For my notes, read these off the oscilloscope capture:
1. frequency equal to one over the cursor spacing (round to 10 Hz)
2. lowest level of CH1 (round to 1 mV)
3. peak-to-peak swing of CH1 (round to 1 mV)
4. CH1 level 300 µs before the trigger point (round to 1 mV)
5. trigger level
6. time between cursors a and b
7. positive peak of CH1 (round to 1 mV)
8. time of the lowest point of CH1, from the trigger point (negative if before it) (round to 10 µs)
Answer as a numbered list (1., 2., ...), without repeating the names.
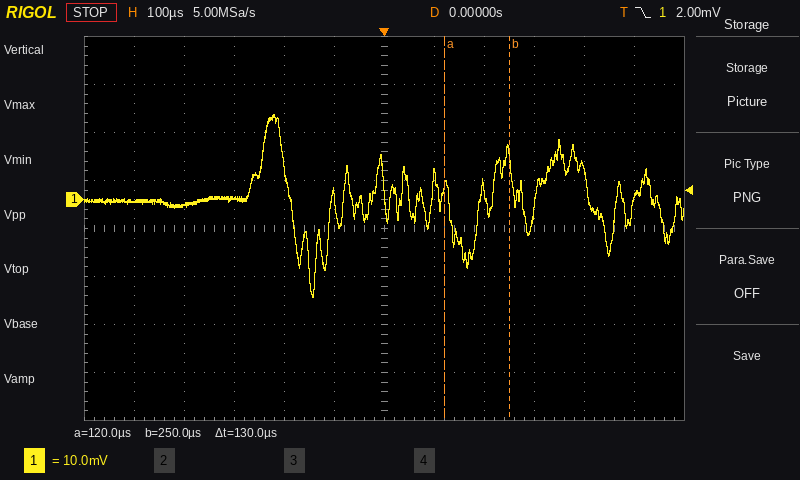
1. 7.69 kHz
2. -20 mV
3. 38 mV
4. 0 mV
5. 2.00 mV
6. 130 µs
7. 18 mV
8. -140 µs
